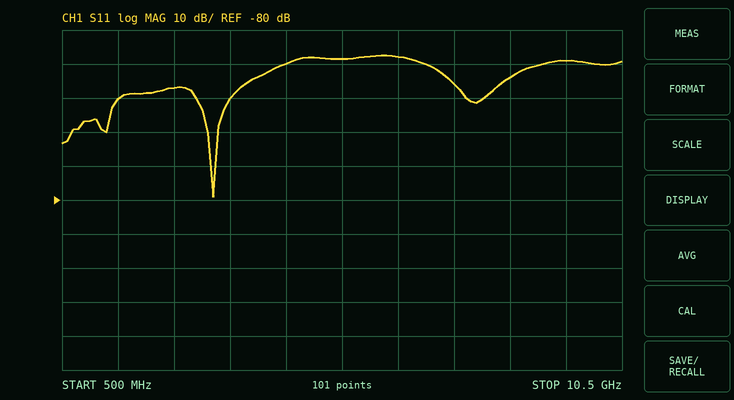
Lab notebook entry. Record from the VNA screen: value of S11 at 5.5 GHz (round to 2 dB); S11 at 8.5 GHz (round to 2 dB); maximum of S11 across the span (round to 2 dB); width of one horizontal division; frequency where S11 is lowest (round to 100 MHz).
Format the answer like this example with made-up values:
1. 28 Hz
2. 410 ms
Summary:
1. -38 dB
2. -44 dB
3. -38 dB
4. 1 GHz
5. 3.2 GHz
